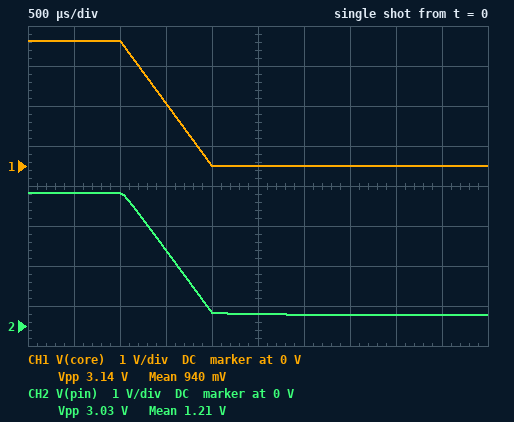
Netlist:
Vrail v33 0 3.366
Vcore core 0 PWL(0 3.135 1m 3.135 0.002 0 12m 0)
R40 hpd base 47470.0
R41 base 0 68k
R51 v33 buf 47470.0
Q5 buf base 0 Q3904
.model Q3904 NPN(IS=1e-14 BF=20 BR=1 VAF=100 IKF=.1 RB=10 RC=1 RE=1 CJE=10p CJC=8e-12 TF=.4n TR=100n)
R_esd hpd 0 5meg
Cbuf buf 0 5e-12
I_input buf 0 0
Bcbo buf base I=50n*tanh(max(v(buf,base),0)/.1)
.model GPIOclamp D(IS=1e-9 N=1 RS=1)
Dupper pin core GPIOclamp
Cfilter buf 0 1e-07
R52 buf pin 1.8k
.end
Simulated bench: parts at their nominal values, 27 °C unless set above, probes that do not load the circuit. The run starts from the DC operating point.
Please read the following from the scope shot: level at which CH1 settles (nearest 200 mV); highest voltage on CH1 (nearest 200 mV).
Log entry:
0 V
3.2 V
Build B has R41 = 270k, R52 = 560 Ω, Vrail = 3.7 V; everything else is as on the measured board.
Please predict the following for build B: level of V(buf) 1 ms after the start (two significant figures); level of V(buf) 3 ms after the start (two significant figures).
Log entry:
3.4 V
330 mV
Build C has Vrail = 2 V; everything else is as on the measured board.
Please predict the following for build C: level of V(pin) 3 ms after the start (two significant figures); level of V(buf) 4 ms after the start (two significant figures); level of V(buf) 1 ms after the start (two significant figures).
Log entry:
270 mV
330 mV
2.0 V
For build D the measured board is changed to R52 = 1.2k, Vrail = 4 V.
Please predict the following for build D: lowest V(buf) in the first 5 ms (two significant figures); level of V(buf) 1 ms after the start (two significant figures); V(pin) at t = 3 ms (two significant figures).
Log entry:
380 mV
3.4 V
290 mV
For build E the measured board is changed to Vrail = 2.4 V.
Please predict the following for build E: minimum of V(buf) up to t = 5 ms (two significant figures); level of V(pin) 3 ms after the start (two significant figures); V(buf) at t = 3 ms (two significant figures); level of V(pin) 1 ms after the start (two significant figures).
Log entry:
350 mV
280 mV
360 mV
2.4 V
